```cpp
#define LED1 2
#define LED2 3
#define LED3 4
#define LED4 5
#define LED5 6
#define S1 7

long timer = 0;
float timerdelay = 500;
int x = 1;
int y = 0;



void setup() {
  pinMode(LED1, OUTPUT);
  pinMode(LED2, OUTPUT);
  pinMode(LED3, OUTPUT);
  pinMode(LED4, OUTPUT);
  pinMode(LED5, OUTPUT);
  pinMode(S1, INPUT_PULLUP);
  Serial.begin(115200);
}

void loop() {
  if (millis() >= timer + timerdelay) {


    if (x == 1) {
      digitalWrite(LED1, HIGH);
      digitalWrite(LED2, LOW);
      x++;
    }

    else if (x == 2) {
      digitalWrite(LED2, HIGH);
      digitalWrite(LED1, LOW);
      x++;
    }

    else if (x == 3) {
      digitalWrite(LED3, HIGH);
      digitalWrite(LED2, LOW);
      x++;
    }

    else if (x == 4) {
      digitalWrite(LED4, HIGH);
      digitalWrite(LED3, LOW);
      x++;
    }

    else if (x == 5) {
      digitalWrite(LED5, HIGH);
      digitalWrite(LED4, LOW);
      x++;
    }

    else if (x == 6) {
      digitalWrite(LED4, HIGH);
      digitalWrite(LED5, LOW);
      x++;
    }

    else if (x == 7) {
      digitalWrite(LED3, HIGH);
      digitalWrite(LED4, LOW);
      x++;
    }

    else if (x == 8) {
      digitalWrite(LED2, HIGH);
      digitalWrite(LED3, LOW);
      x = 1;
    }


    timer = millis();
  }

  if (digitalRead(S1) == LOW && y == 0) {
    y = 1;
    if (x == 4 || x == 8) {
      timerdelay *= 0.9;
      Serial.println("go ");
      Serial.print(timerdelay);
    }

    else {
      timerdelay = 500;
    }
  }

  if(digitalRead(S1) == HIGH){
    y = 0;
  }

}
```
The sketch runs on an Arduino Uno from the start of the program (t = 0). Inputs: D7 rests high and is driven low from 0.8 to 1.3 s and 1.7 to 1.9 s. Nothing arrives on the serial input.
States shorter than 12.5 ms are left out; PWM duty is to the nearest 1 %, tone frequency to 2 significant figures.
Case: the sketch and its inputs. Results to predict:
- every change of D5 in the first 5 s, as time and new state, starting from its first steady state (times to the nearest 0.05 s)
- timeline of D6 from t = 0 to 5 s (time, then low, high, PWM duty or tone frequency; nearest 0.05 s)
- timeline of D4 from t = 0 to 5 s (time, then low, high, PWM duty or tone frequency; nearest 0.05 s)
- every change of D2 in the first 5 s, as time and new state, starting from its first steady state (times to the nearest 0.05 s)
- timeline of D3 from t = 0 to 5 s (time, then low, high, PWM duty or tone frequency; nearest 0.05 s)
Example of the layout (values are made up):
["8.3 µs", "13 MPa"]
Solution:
["0 s low; 1.95 s high; 2.4 s low; 2.85 s high; 3.3 s low", "0 s low; 2.4 s high; 2.85 s low", "0 s low; 1.5 s high; 1.95 s low; 3.3 s high; 3.75 s low", "0 s low; 0.5 s high; 1 s low; 4.2 s high; 4.65 s low", "0 s low; 1 s high; 1.5 s low; 3.75 s high; 4.2 s low; 4.65 s high"]
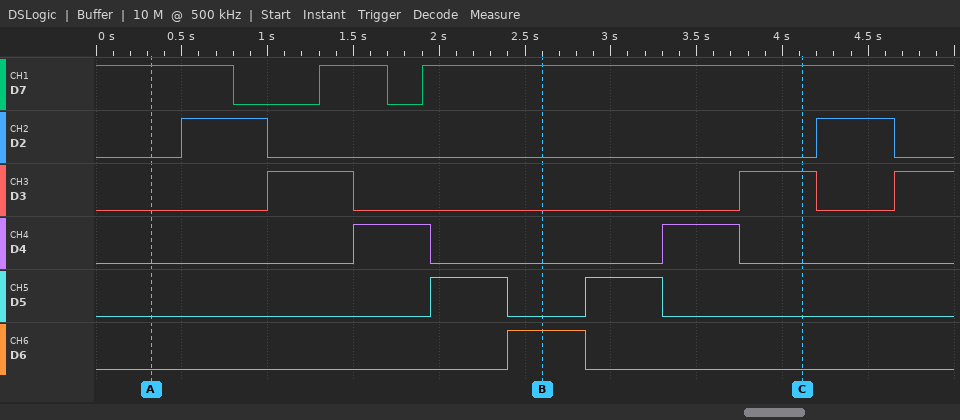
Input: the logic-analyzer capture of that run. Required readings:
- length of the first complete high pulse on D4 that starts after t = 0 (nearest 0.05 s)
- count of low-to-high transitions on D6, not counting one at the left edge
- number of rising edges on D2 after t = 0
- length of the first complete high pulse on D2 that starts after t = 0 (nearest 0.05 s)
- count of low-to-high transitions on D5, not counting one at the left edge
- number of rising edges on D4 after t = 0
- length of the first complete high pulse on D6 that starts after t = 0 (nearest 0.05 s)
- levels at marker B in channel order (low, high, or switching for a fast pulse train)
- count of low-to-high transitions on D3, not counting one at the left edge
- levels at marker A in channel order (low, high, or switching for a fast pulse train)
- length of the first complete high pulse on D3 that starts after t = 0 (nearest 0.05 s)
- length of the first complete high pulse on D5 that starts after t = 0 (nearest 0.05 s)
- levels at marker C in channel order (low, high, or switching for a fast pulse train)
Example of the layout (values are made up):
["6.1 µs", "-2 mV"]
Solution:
["0.45 s", "1", "2", "0.50 s", "2", "2", "0.45 s", "D7 high, D2 low, D3 low, D4 low, D5 low, D6 high", "3", "D7 high, D2 low, D3 low, D4 low, D5 low, D6 low", "0.50 s", "0.45 s", "D7 high, D2 low, D3 high, D4 low, D5 low, D6 low"]
